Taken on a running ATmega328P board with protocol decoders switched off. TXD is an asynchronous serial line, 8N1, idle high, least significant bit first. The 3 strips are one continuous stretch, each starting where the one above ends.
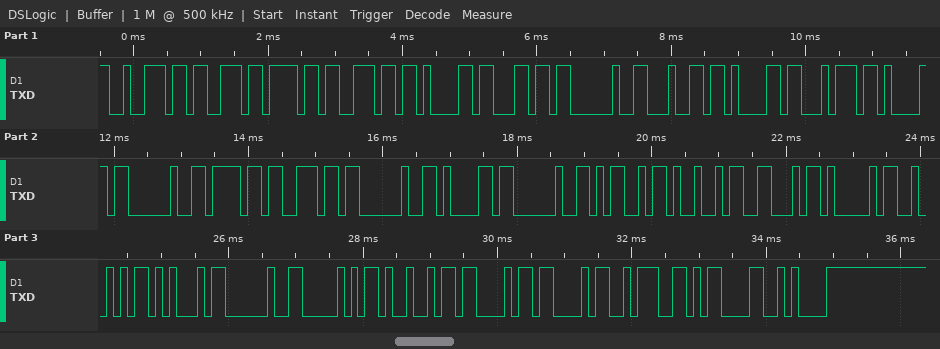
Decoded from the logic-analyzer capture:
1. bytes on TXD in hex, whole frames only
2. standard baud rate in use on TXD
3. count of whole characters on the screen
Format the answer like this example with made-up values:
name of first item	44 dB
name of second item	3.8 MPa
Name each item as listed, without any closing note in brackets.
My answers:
bytes on TXD in hex, whole frames only	72 73 6F 6E 61 6C 20 64 61 74 61 20 6F 6E 20 61 20 4D 49 46 41 52 45 20 50 49 43 43 3A 0D 0A
standard baud rate in use on TXD	9600 baud
count of whole characters on the screen	31
